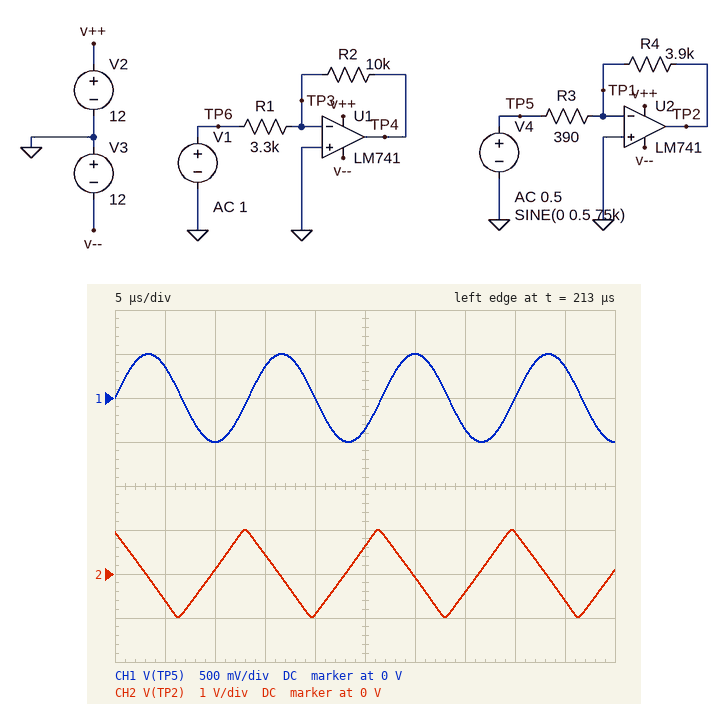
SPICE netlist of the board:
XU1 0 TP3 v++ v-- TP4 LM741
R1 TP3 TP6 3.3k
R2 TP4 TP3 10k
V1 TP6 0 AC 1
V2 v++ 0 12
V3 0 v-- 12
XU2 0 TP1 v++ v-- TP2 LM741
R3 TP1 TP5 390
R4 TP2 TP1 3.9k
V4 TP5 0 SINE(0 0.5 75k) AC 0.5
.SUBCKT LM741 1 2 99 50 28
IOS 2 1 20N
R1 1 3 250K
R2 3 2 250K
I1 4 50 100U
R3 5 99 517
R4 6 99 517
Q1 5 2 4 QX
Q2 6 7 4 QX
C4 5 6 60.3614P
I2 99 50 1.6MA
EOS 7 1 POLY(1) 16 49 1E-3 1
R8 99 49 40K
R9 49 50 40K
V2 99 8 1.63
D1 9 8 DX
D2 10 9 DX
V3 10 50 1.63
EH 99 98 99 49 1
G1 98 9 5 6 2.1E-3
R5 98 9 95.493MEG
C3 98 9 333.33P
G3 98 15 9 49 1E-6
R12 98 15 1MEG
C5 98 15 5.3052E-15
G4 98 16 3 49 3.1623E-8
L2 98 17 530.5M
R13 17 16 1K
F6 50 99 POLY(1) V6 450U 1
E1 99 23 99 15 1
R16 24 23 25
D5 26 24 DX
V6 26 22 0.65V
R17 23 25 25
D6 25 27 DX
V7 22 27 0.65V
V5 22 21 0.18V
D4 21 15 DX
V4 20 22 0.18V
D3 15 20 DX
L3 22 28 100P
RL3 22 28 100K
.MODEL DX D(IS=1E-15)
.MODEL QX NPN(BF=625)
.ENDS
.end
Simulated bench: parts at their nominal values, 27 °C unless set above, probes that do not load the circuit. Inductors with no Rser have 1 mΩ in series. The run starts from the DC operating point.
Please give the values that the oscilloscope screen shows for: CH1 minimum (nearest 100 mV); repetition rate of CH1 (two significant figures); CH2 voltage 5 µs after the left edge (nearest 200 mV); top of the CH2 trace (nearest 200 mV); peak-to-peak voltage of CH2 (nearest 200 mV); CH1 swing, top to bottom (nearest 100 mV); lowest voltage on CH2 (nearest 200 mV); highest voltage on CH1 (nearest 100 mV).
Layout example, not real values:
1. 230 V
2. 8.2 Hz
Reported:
1. -500 mV
2. 75 kHz
3. -600 mV
4. 1.0 V
5. 2.0 V
6. 1.0 V
7. -1.0 V
8. 500 mV
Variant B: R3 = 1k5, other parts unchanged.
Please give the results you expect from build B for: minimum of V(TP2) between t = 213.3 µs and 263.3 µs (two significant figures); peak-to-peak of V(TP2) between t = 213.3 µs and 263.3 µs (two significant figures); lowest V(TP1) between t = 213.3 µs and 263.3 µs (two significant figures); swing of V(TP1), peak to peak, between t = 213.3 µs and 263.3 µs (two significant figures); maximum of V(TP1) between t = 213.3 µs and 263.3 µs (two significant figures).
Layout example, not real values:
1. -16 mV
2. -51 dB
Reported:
1. -950 mV
2. 1.9 V
3. -270 mV
4. 550 mV
5. 270 mV
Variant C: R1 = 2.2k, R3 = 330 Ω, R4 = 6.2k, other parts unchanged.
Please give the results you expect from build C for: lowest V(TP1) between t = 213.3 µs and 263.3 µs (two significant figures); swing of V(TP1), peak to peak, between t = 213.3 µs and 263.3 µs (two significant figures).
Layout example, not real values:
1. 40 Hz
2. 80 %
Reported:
1. -470 mV
2. 950 mV
